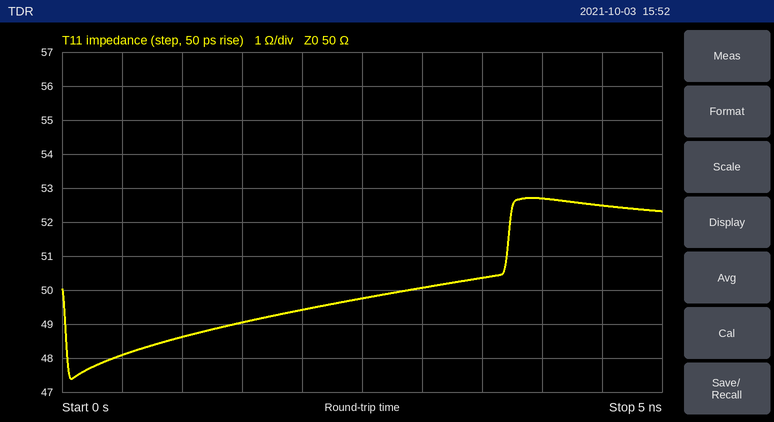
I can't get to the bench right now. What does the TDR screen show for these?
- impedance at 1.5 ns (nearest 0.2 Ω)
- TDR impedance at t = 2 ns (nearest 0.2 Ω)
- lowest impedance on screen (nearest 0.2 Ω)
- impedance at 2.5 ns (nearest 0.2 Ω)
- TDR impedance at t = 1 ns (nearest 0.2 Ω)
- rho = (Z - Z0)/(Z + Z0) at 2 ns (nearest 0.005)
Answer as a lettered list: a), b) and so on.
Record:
a) 49.0 Ω
b) 49.4 Ω
c) 47.4 Ω
d) 49.8 Ω
e) 48.6 Ω
f) -0.005
